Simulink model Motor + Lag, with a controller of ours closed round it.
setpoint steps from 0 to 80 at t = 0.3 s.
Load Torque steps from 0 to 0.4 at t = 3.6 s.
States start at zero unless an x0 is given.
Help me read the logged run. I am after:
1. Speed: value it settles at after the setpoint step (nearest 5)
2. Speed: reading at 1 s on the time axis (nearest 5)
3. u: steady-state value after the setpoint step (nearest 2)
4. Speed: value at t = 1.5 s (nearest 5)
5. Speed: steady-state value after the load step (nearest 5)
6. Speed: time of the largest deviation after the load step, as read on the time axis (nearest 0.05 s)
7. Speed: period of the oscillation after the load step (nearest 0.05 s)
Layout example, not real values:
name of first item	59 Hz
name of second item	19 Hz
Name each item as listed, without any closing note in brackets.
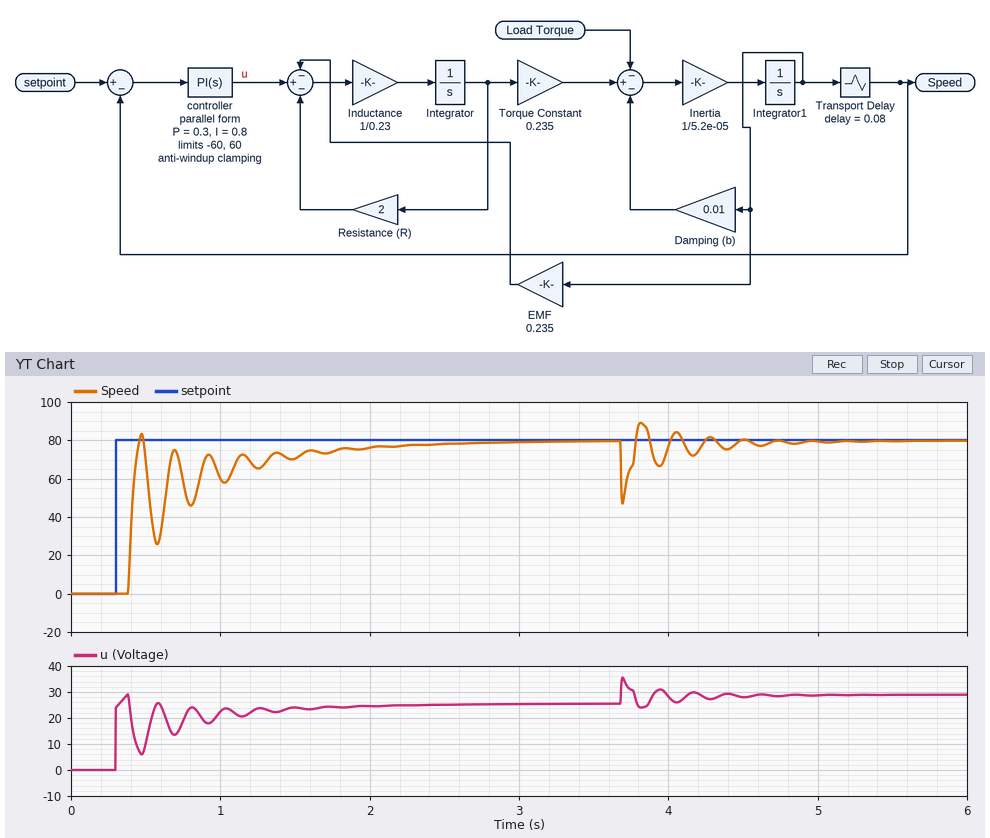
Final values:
Speed: value it settles at after the setpoint step	80
Speed: reading at 1 s on the time axis	60
u: steady-state value after the setpoint step	26
Speed: value at t = 1.5 s	70
Speed: steady-state value after the load step	80
Speed: time of the largest deviation after the load step, as read on the time axis	3.70 s
Speed: period of the oscillation after the load step	0.25 s
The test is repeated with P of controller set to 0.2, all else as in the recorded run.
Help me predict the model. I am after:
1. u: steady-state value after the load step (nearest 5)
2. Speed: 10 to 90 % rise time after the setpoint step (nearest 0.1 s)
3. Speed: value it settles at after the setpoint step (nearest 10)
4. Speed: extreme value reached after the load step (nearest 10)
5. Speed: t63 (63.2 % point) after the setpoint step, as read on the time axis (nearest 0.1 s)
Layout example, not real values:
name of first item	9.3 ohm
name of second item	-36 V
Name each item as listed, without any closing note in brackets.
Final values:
u: steady-state value after the load step	30
Speed: 10 to 90 % rise time after the setpoint step	1.0 s
Speed: value it settles at after the setpoint step	80
Speed: extreme value reached after the load step	50
Speed: t63 (63.2 % point) after the setpoint step, as read on the time axis	0.4 s
